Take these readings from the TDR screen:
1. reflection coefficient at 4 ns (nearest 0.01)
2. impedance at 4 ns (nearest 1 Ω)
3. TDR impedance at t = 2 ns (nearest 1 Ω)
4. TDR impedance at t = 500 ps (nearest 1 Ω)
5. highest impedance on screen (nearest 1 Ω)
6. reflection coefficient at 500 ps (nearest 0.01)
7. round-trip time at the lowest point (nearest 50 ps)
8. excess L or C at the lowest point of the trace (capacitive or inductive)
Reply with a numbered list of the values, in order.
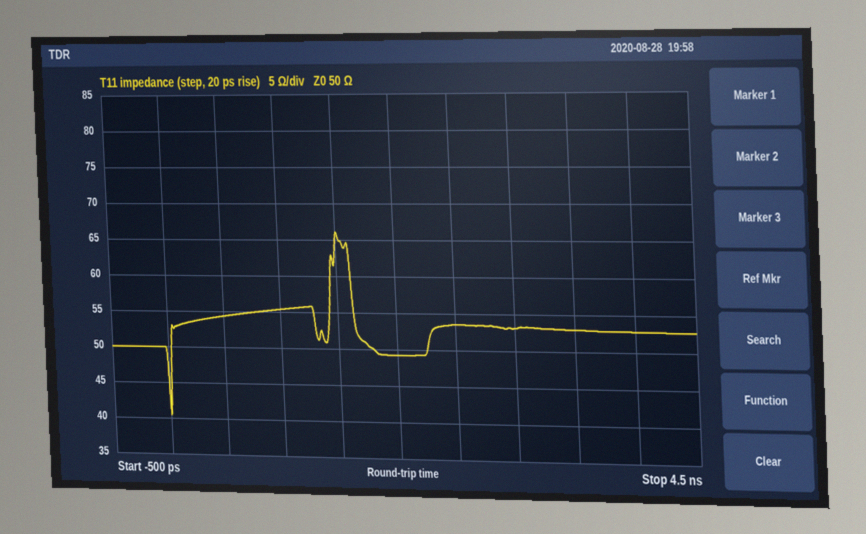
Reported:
1. +0.03
2. 53 Ω
3. 49 Ω
4. 54 Ω
5. 66 Ω
6. +0.04
7. 0 ps
8. capacitive
